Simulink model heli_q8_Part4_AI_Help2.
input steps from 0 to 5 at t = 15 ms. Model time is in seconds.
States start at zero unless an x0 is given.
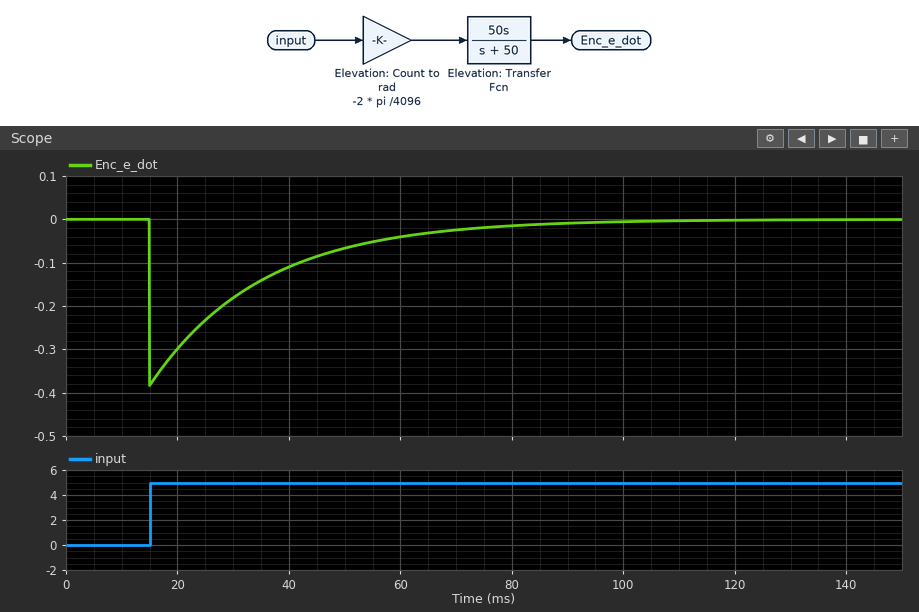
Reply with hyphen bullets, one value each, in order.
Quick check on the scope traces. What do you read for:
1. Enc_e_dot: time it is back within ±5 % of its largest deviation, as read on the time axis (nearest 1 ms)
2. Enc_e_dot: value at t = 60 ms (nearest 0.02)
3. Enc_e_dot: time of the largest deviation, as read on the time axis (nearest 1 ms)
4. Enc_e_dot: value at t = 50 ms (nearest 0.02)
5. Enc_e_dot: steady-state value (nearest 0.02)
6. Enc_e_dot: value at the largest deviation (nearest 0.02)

- 75 ms
- -0.04
- 15 ms
- -0.06
- 0.00
- -0.38
